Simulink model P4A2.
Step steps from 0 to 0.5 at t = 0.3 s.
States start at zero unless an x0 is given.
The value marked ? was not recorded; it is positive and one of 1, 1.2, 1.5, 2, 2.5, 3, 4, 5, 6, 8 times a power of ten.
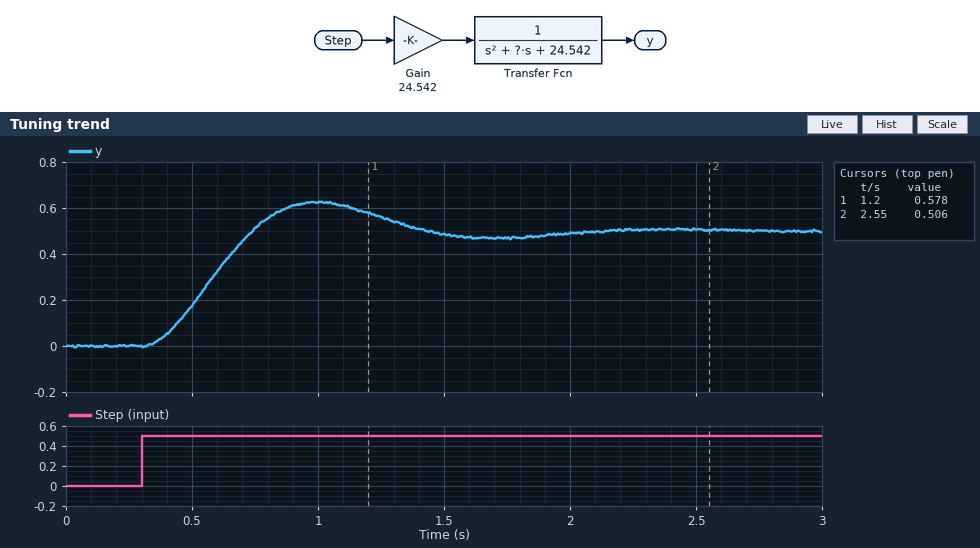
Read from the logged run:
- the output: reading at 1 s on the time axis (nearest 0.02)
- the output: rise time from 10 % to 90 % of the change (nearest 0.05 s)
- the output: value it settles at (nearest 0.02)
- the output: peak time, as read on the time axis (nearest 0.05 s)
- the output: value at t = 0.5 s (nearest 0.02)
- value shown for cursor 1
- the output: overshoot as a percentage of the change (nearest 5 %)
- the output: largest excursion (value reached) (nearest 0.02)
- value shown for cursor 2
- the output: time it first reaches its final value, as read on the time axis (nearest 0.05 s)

0.62
0.30 s
0.50
1.00 s
0.18
0.578
25 %
0.62
0.506
0.75 s
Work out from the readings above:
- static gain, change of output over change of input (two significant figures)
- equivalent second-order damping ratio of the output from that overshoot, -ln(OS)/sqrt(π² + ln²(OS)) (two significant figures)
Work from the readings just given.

1.0
0.40
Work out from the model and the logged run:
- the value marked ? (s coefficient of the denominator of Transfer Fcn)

4
